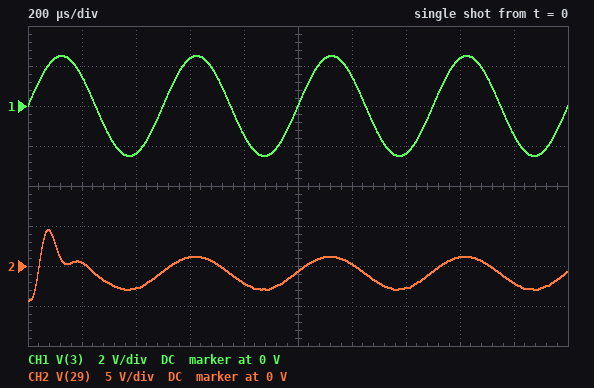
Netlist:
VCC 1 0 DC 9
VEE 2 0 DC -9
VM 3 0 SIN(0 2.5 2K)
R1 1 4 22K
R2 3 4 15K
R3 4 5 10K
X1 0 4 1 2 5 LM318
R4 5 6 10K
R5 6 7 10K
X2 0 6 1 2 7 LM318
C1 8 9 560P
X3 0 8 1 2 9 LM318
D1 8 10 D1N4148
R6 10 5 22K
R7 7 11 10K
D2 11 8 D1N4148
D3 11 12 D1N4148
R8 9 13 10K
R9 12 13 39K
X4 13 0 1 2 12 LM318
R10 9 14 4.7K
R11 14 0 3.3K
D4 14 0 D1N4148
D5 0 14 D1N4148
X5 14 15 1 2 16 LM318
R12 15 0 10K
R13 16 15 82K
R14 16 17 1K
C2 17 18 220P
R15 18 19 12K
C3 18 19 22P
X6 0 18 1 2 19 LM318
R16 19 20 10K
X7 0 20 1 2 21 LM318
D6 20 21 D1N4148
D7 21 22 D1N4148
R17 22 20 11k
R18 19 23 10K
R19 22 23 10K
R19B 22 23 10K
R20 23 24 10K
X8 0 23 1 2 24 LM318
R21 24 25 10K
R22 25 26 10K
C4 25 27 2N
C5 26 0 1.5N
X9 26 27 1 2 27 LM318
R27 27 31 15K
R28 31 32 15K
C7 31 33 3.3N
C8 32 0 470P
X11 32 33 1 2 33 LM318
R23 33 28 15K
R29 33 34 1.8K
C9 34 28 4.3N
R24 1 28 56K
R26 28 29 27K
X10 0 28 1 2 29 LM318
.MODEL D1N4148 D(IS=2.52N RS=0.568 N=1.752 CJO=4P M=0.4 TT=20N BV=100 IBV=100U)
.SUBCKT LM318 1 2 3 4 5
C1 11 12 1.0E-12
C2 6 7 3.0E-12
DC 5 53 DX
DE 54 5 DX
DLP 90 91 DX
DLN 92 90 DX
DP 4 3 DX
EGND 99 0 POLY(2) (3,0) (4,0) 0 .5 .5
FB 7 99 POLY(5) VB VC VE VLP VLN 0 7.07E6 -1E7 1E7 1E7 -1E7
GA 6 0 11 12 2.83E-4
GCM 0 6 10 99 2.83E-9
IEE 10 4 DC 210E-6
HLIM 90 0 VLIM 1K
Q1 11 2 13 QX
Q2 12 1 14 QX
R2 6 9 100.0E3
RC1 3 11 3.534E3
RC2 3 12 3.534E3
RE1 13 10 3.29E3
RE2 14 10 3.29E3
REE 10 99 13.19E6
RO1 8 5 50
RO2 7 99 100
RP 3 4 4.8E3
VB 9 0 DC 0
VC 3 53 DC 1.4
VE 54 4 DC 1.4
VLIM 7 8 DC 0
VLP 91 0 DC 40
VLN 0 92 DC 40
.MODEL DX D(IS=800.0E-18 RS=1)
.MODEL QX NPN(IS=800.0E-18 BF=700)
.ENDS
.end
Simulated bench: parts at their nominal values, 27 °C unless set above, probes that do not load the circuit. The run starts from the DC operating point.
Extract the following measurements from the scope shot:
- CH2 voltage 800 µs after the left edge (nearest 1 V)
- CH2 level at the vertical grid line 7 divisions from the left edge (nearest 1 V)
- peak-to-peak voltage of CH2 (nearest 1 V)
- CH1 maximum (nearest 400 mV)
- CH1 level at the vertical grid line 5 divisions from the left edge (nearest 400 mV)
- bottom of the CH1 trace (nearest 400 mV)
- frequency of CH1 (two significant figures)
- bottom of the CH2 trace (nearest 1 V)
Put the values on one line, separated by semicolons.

-2 V; -3 V; 9 V; 2.4 V; 0 V; -2.4 V; 2.0 kHz; -4 V
